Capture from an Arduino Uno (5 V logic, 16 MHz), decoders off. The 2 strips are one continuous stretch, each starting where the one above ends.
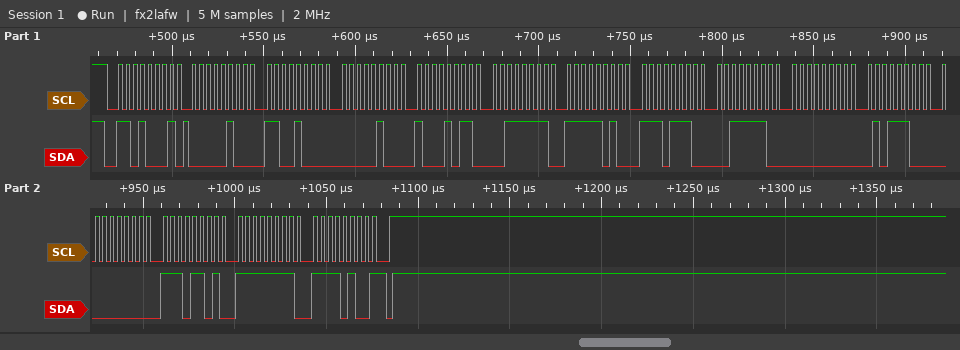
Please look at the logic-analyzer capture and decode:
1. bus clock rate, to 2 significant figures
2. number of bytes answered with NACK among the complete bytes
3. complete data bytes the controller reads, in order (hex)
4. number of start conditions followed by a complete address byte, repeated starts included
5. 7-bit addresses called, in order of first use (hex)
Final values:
250 kHz
1
04 C8 04 8B 3F FA EE 3E 00 5C 00 ED FF F4
1
0x68
